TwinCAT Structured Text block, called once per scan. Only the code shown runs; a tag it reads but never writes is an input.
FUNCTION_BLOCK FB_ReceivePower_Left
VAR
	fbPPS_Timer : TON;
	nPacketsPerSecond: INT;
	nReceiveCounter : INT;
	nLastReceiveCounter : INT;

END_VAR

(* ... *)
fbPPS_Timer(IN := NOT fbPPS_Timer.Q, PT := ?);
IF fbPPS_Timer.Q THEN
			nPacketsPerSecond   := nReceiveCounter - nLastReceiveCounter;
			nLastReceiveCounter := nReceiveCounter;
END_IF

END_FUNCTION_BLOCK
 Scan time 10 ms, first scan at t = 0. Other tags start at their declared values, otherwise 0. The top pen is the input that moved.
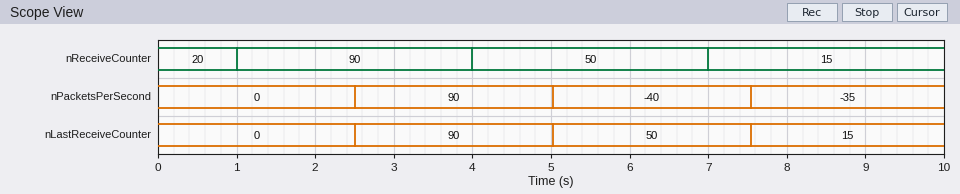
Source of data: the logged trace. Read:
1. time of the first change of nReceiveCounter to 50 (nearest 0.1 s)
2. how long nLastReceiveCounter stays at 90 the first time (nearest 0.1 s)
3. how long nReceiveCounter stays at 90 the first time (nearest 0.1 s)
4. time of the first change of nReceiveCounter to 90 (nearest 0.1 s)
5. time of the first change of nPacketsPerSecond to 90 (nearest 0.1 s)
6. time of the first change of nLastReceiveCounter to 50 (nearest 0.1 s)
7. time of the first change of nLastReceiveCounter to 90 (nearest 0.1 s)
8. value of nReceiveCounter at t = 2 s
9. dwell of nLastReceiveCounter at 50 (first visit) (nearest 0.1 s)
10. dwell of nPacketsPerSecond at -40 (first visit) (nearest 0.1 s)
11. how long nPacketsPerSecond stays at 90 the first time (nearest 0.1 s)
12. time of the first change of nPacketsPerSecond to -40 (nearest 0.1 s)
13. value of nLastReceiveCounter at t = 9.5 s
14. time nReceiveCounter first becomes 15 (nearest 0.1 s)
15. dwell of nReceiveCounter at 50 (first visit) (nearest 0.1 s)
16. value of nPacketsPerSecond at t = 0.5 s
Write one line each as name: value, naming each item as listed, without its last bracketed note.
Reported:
time of the first change of nReceiveCounter to 50: 4.0 s
how long nLastReceiveCounter stays at 90 the first time: 2.5 s
how long nReceiveCounter stays at 90 the first time: 3.0 s
time of the first change of nReceiveCounter to 90: 1.0 s
time of the first change of nPacketsPerSecond to 90: 2.5 s
time of the first change of nLastReceiveCounter to 50: 5.0 s
time of the first change of nLastReceiveCounter to 90: 2.5 s
value of nReceiveCounter at t = 2 s: 90
dwell of nLastReceiveCounter at 50 (first visit): 2.5 s
dwell of nPacketsPerSecond at -40 (first visit): 2.5 s
how long nPacketsPerSecond stays at 90 the first time: 2.5 s
time of the first change of nPacketsPerSecond to -40: 5.0 s
value of nLastReceiveCounter at t = 9.5 s: 15
time nReceiveCounter first becomes 15: 7.0 s
dwell of nReceiveCounter at 50 (first visit): 3.0 s
value of nPacketsPerSecond at t = 0.5 s: 0
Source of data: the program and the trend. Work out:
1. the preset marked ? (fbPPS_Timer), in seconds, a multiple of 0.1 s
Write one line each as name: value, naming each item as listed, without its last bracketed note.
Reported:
the preset marked ? (fbPPS_Timer), in seconds, a multiple of 0.1 s: 2.5 s
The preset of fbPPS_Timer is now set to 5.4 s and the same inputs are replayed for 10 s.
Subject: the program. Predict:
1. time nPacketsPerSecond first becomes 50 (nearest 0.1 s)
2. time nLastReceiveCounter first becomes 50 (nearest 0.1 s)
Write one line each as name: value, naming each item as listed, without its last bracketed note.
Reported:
time nPacketsPerSecond first becomes 50: 5.4 s
time nLastReceiveCounter first becomes 50: 5.4 s
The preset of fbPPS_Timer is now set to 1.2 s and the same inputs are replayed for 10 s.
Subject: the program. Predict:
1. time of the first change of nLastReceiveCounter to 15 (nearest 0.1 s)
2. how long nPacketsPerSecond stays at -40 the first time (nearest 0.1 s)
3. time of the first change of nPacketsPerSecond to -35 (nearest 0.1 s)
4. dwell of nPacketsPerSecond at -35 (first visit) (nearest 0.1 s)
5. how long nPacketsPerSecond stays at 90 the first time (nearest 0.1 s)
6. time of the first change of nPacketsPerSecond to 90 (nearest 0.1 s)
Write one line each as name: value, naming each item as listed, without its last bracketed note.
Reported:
time of the first change of nLastReceiveCounter to 15: 7.3 s
how long nPacketsPerSecond stays at -40 the first time: 1.2 s
time of the first change of nPacketsPerSecond to -35: 7.3 s
dwell of nPacketsPerSecond at -35 (first visit): 1.2 s
how long nPacketsPerSecond stays at 90 the first time: 1.2 s
time of the first change of nPacketsPerSecond to 90: 1.2 s
